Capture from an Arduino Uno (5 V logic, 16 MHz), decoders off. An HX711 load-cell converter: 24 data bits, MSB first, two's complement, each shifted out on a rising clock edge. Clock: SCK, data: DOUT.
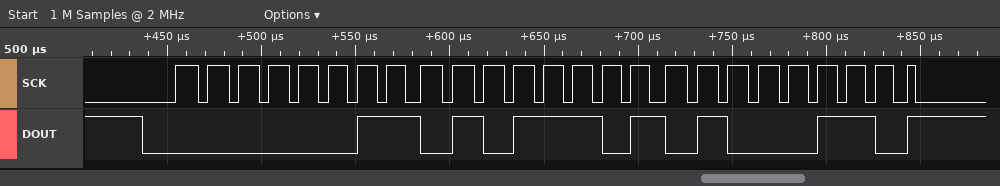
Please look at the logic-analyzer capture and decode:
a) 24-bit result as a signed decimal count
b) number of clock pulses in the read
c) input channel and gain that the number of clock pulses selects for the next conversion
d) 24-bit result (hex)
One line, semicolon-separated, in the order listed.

220486; 25; channel A, gain 128; 0x035D46
